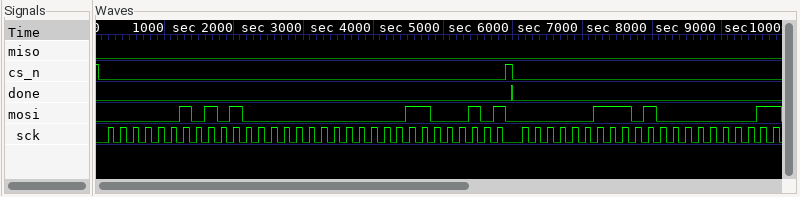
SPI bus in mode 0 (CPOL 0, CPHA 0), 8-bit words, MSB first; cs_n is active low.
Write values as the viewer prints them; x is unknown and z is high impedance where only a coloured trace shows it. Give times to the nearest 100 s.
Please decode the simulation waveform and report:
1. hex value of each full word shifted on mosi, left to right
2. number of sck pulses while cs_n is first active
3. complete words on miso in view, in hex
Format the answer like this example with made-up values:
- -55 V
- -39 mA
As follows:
- 02, A0, 00, C5, 03, A0
- 32
- 00, 00, 00, 00, 00, 00
